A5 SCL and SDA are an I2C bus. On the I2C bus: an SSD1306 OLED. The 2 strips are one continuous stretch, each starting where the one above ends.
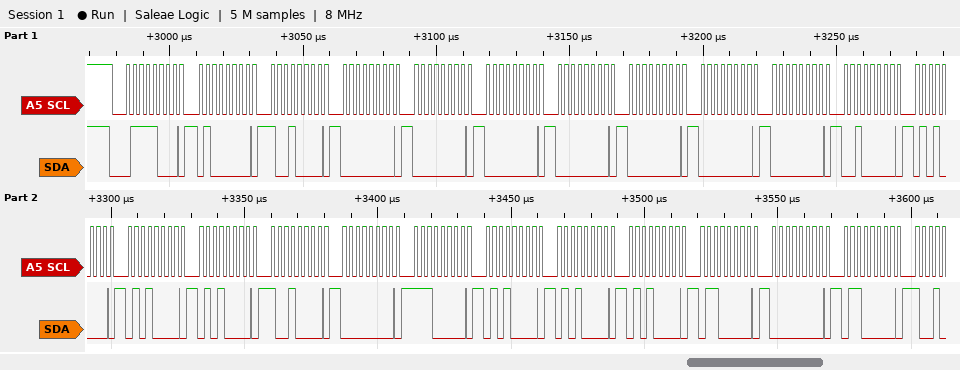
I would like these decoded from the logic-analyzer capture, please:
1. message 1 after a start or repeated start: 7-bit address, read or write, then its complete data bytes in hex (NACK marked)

0x3C write: 40 90 00 00 00 00 00 00 00 20 50 50 50 90 00 E0 50 50 50 60 00 60
